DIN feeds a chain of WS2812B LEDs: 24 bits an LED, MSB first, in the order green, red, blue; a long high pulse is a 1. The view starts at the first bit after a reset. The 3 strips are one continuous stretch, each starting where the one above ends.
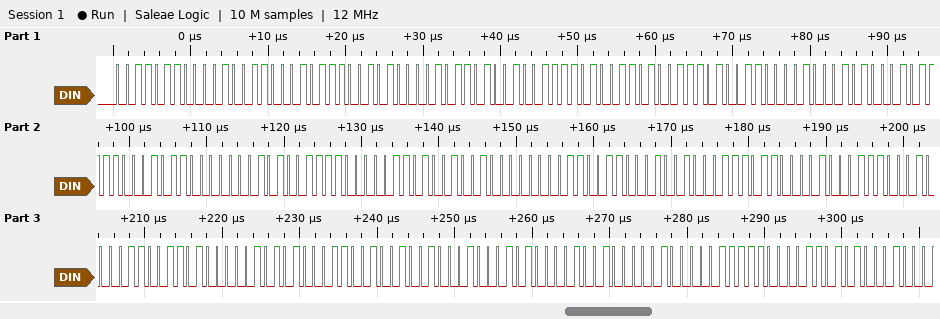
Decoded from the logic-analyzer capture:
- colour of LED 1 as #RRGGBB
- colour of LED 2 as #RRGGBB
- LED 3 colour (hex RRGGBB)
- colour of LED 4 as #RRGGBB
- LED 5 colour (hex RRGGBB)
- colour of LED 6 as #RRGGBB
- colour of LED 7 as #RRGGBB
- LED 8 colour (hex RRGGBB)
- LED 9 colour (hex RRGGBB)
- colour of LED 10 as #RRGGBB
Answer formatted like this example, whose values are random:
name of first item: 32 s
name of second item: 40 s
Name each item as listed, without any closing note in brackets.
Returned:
colour of LED 1 as #RRGGBB: #133617
colour of LED 2 as #RRGGBB: #5A284F
LED 3 colour: #3A4D61
colour of LED 4 as #RRGGBB: #5E142C
LED 5 colour: #3C051A
colour of LED 6 as #RRGGBB: #064862
colour of LED 7 as #RRGGBB: #61471C
LED 8 colour: #344315
LED 9 colour: #241945
colour of LED 10 as #RRGGBB: #04091F
